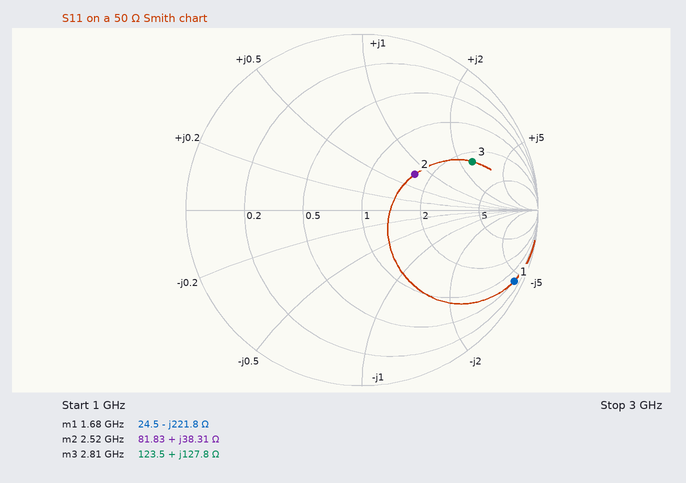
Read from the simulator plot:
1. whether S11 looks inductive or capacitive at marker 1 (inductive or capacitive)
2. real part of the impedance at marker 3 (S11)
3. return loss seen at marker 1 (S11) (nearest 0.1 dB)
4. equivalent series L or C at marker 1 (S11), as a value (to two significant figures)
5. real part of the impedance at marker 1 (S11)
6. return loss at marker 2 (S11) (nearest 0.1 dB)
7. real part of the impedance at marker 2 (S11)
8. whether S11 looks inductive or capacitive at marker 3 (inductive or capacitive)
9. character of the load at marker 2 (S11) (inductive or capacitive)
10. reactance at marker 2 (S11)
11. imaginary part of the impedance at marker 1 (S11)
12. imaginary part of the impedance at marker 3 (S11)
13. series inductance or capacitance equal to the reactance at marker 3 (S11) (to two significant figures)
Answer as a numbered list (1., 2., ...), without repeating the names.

1. capacitive
2. 123.5 Ω
3. 0.4 dB
4. 430 fF
5. 24.5 Ω
6. 8.8 dB
7. 81.83 Ω
8. inductive
9. inductive
10. +38.31 Ω
11. -221.8 Ω
12. +127.8 Ω
13. 7.2 nH
